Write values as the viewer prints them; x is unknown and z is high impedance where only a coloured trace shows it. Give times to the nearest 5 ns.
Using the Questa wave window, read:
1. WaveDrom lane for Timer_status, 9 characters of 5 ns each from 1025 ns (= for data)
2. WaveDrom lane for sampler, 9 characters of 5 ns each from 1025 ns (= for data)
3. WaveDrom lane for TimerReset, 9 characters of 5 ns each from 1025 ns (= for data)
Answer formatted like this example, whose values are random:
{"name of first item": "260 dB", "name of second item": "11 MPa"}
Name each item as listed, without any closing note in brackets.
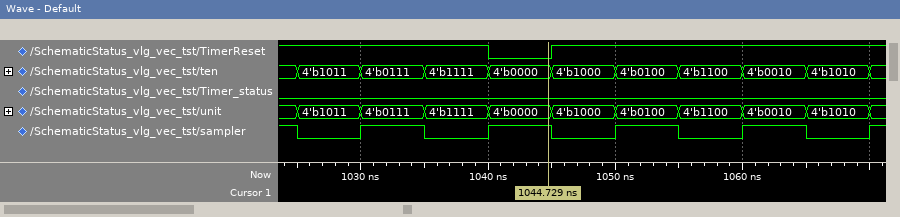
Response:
{"WaveDrom lane for Timer_status, 9 characters of 5 ns each from 1025 ns": "{name: 'Timer_status', wave: '0........'}", "WaveDrom lane for sampler, 9 characters of 5 ns each from 1025 ns": "{name: 'sampler', wave: '010101010'}", "WaveDrom lane for TimerReset, 9 characters of 5 ns each from 1025 ns": "{name: 'TimerReset', wave: '1..01....'}"}
